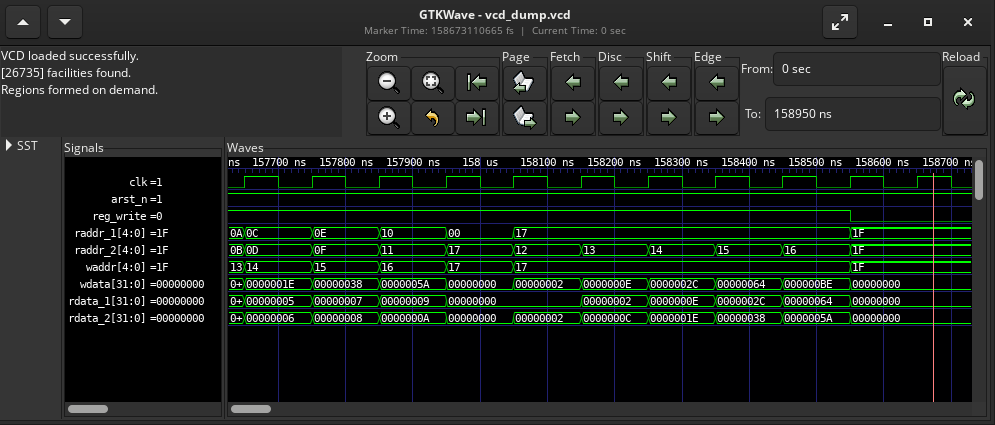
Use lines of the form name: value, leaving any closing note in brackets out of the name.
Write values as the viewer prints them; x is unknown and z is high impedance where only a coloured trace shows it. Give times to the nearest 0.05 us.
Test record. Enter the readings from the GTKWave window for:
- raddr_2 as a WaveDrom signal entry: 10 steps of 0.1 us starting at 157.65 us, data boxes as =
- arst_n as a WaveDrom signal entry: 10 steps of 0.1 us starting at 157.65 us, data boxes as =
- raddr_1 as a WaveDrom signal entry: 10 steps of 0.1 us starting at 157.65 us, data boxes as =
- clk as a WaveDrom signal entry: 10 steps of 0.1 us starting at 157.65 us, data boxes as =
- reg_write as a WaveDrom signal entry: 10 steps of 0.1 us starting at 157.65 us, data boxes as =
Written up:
raddr_2 as a WaveDrom signal entry: 10 steps of 0.1 us starting at 157.65 us, data boxes as =: {name: 'raddr_2', wave: '==========', data: '0D 0F 11 17 12 13 14 15 16 1F'}
arst_n as a WaveDrom signal entry: 10 steps of 0.1 us starting at 157.65 us, data boxes as =: {name: 'arst_n', wave: '1.........'}
raddr_1 as a WaveDrom signal entry: 10 steps of 0.1 us starting at 157.65 us, data boxes as =: {name: 'raddr_1', wave: '=====....=', data: '0C 0E 10 00 17 1F'}
clk as a WaveDrom signal entry: 10 steps of 0.1 us starting at 157.65 us, data boxes as =: {name: 'clk', wave: 'p.........'}
reg_write as a WaveDrom signal entry: 10 steps of 0.1 us starting at 157.65 us, data boxes as =: {name: 'reg_write', wave: '1........0'}
